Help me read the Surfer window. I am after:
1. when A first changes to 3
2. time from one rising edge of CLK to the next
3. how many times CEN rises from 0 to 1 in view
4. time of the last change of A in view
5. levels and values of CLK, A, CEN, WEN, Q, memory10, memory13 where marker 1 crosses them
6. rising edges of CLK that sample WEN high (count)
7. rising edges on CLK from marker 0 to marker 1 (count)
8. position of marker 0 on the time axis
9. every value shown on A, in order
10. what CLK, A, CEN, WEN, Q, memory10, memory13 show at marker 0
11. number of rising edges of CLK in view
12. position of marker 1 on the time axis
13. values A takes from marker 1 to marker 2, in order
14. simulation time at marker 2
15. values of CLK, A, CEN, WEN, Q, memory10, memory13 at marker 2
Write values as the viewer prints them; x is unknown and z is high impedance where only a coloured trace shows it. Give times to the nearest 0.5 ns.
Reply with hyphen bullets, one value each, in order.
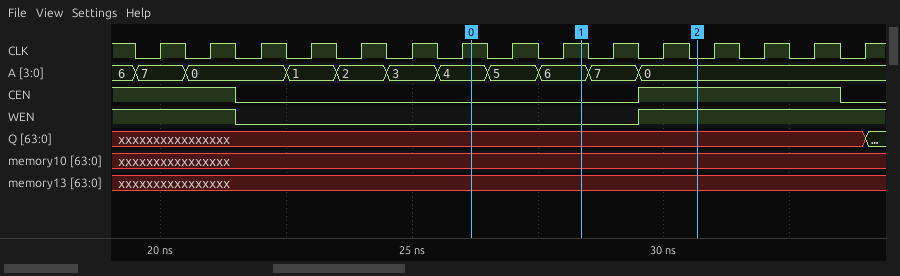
- 24.5 ns
- 1 ns
- 1
- 29.5 ns
- CLK=1, A=6, CEN=0, WEN=0, Q=xxxxxxxxxxxxxxxx, memory10=xxxxxxxxxxxxxxxx, memory13=xxxxxxxxxxxxxxxx
- 7
- 2
- 26 ns
- 6, 7, 0, 1, 2, 3, 4, 5, 6, 7, 0
- CLK=1, A=4, CEN=0, WEN=0, Q=xxxxxxxxxxxxxxxx, memory10=xxxxxxxxxxxxxxxx, memory13=xxxxxxxxxxxxxxxx
- 15
- 28.5 ns
- 6, 7, 0
- 30.5 ns
- CLK=0, A=0, CEN=1, WEN=1, Q=xxxxxxxxxxxxxxxx, memory10=xxxxxxxxxxxxxxxx, memory13=xxxxxxxxxxxxxxxx
